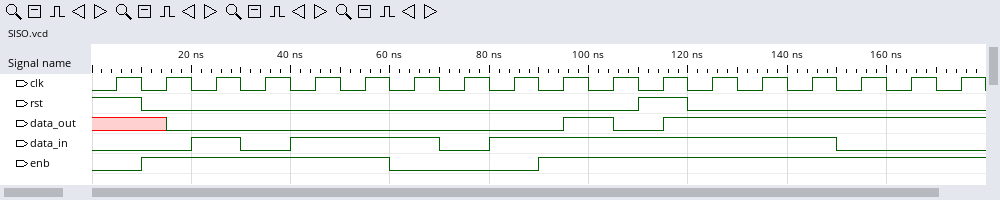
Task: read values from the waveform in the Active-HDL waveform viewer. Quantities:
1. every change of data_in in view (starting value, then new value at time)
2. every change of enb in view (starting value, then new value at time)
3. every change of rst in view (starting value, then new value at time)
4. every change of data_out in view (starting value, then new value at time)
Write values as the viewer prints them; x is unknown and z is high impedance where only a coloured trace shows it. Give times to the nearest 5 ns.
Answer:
0, 1 at 20 ns, 0 at 30 ns, 1 at 40 ns, 0 at 70 ns, 1 at 80 ns, 0 at 150 ns
0, 1 at 10 ns, 0 at 60 ns, 1 at 90 ns
1, 0 at 10 ns, 1 at 110 ns, 0 at 120 ns
x, 0 at 15 ns, 1 at 95 ns, 0 at 105 ns, 1 at 115 ns
